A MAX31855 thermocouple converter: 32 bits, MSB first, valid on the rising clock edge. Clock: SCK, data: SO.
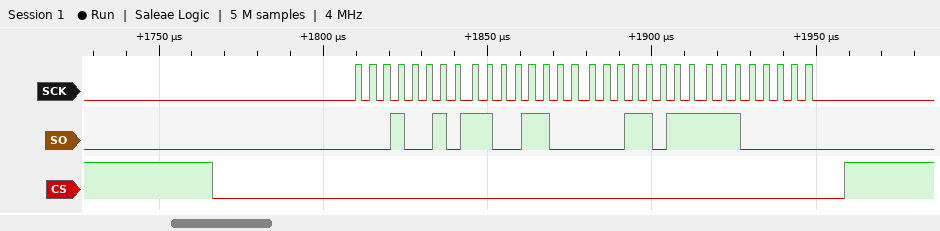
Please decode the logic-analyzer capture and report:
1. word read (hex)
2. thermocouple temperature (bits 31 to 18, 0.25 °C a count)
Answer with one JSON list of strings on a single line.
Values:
["0x12CC1BE0", "300.75 °C"]
